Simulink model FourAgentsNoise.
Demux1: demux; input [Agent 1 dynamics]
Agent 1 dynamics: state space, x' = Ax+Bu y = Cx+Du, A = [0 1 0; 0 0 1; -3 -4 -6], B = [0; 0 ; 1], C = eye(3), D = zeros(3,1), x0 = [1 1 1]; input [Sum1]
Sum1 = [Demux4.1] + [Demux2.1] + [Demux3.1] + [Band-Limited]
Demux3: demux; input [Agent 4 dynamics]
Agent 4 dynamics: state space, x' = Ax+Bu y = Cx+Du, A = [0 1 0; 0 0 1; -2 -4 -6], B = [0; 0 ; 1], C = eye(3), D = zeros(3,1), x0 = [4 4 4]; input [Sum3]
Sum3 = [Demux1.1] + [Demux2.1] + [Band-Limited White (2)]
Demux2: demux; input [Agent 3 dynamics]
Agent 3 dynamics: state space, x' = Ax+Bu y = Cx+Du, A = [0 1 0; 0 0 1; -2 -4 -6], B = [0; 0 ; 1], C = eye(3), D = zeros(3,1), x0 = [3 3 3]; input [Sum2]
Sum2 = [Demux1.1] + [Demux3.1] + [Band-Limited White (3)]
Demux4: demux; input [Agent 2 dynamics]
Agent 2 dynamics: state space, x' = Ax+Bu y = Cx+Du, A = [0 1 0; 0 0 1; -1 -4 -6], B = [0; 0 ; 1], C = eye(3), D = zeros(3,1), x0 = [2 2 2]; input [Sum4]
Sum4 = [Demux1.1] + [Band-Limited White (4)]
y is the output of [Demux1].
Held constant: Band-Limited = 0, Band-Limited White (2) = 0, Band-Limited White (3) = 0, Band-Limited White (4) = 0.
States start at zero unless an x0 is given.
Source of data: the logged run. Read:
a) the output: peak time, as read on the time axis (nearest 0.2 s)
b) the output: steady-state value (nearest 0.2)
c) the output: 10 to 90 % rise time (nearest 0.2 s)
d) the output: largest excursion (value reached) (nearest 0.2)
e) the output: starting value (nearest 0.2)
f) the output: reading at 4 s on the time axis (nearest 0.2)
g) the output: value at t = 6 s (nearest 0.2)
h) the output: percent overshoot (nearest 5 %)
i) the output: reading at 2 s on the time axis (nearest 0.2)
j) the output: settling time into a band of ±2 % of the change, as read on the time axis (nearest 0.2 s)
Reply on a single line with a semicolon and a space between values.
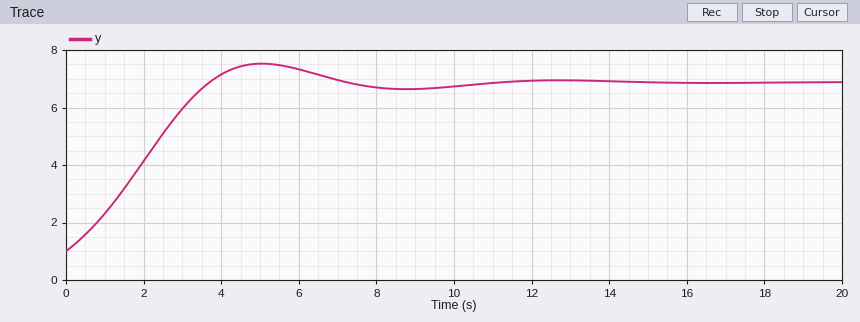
5.0 s; 6.8; 2.8 s; 7.6; 1.0; 7.2; 7.4; 10 %; 4.2; 10.2 s
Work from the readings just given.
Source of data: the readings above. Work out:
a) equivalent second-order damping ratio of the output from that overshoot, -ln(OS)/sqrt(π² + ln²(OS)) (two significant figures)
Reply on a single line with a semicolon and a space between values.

0.59
